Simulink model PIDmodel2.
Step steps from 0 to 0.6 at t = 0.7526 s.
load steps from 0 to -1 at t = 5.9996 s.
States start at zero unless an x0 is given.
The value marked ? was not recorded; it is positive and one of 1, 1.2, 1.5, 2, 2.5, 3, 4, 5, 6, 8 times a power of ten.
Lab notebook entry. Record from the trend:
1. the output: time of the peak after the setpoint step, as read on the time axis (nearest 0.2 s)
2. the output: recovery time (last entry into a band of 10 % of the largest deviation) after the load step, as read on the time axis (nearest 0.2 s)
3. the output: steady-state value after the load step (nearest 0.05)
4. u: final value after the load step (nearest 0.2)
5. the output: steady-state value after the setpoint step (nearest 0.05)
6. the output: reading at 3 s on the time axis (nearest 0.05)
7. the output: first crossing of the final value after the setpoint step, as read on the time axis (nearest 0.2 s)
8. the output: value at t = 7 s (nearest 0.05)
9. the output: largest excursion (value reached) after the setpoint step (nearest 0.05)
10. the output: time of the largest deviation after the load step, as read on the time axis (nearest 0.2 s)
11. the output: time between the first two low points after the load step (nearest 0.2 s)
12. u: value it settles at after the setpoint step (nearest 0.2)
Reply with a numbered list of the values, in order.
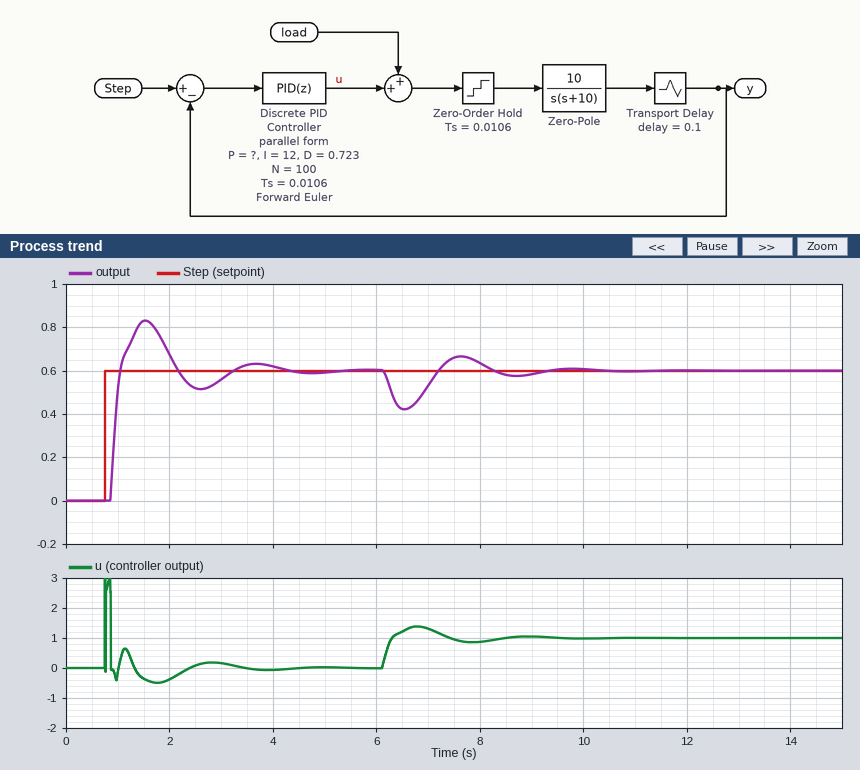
1. 1.6 s
2. 9.0 s
3. 0.60
4. 1.0
5. 0.60
6. 0.55
7. 1.0 s
8. 0.55
9. 0.85
10. 6.6 s
11. 2.2 s
12. 0.0
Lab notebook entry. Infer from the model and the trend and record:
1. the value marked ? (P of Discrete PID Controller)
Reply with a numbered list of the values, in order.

1. 4
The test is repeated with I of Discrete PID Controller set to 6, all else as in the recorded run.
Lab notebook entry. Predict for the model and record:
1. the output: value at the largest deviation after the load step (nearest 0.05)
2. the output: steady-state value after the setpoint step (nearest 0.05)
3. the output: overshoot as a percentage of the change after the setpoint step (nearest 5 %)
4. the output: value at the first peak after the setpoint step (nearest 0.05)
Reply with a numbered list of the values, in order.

1. 0.40
2. 0.60
3. 20 %
4. 0.75
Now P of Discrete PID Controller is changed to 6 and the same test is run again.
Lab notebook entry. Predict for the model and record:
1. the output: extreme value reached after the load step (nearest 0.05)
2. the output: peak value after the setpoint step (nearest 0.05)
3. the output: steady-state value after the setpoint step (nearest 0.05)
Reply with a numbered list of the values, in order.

1. 0.45
2. 0.80
3. 0.60
